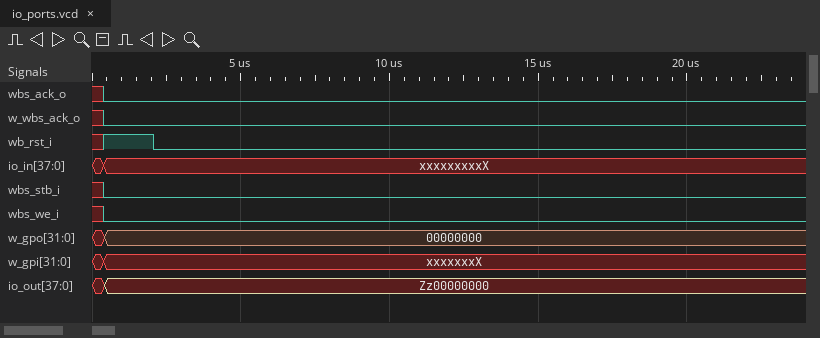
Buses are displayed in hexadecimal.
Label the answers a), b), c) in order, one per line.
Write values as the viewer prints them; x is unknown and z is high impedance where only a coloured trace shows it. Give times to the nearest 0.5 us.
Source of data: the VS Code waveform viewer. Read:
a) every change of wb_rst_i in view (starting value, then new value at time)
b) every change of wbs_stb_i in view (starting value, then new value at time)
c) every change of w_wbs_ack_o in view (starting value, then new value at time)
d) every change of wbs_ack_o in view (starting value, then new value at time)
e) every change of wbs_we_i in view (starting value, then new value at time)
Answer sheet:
a) x, 1 at 0.5 us, 0 at 2 us
b) x, 0 at 0.5 us
c) x, 0 at 0.5 us
d) x, 0 at 0.5 us
e) x, 0 at 0.5 us
